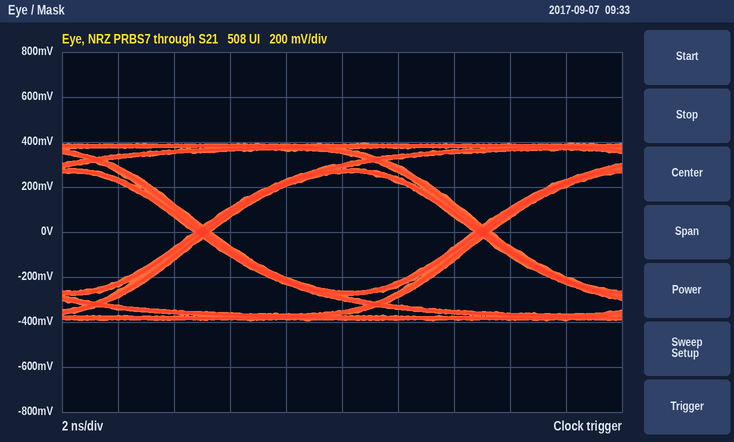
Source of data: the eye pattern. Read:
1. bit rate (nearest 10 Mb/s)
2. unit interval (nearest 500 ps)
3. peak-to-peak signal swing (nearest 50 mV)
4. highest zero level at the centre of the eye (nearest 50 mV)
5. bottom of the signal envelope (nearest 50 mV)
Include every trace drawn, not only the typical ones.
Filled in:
100 Mb/s
10.0 ns
800 mV
-250 mV
-400 mV
